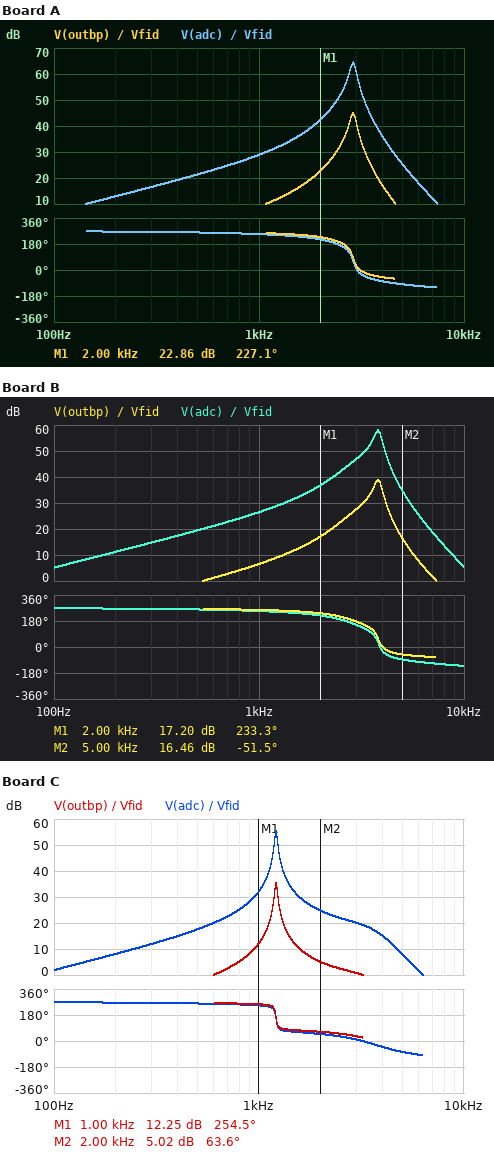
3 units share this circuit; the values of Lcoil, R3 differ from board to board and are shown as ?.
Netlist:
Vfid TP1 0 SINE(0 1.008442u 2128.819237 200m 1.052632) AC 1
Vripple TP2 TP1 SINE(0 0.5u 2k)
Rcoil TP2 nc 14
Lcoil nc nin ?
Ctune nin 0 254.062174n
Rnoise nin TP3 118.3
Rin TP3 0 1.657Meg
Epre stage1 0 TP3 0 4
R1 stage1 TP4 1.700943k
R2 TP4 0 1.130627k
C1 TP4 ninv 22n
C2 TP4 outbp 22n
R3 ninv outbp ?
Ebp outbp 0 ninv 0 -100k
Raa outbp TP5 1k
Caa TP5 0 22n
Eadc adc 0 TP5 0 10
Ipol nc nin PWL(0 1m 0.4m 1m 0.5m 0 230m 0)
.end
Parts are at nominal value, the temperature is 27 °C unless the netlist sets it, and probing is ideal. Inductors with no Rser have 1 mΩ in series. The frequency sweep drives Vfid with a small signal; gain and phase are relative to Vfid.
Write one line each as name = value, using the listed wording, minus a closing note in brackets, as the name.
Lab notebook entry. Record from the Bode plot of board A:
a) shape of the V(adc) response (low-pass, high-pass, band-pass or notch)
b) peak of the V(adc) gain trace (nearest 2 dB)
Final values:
shape of the V(adc) response = band-pass
peak of the V(adc) gain trace = 64 dB
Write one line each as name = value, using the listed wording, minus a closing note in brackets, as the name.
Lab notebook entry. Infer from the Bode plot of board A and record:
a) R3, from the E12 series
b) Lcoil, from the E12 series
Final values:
R3, from the E12 series = 10 kΩ
Lcoil, from the E12 series = 12 mH
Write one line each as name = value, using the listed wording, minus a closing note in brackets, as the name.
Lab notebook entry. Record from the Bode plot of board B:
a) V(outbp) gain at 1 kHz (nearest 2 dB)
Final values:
V(outbp) gain at 1 kHz = 6 dB
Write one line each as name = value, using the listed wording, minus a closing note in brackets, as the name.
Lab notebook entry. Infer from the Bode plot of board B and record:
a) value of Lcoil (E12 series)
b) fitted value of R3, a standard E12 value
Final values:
value of Lcoil = 6.8 mH
fitted value of R3, a standard E12 value = 8.2 kΩ
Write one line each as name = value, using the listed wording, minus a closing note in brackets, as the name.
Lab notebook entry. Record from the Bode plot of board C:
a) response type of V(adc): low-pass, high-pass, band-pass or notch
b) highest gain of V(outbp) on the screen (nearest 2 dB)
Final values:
response type of V(adc): low-pass, high-pass, band-pass or notch = band-pass
highest gain of V(outbp) on the screen = 36 dB
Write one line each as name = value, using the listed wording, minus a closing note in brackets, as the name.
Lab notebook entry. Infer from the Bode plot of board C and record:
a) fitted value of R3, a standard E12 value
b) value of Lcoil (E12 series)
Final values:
fitted value of R3, a standard E12 value = 5.6 kΩ
value of Lcoil = 68 mH
